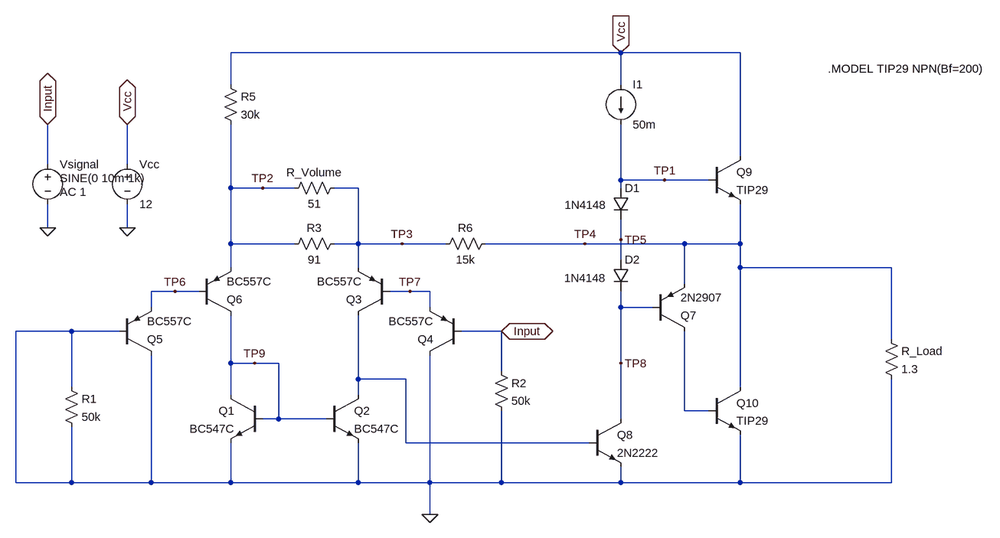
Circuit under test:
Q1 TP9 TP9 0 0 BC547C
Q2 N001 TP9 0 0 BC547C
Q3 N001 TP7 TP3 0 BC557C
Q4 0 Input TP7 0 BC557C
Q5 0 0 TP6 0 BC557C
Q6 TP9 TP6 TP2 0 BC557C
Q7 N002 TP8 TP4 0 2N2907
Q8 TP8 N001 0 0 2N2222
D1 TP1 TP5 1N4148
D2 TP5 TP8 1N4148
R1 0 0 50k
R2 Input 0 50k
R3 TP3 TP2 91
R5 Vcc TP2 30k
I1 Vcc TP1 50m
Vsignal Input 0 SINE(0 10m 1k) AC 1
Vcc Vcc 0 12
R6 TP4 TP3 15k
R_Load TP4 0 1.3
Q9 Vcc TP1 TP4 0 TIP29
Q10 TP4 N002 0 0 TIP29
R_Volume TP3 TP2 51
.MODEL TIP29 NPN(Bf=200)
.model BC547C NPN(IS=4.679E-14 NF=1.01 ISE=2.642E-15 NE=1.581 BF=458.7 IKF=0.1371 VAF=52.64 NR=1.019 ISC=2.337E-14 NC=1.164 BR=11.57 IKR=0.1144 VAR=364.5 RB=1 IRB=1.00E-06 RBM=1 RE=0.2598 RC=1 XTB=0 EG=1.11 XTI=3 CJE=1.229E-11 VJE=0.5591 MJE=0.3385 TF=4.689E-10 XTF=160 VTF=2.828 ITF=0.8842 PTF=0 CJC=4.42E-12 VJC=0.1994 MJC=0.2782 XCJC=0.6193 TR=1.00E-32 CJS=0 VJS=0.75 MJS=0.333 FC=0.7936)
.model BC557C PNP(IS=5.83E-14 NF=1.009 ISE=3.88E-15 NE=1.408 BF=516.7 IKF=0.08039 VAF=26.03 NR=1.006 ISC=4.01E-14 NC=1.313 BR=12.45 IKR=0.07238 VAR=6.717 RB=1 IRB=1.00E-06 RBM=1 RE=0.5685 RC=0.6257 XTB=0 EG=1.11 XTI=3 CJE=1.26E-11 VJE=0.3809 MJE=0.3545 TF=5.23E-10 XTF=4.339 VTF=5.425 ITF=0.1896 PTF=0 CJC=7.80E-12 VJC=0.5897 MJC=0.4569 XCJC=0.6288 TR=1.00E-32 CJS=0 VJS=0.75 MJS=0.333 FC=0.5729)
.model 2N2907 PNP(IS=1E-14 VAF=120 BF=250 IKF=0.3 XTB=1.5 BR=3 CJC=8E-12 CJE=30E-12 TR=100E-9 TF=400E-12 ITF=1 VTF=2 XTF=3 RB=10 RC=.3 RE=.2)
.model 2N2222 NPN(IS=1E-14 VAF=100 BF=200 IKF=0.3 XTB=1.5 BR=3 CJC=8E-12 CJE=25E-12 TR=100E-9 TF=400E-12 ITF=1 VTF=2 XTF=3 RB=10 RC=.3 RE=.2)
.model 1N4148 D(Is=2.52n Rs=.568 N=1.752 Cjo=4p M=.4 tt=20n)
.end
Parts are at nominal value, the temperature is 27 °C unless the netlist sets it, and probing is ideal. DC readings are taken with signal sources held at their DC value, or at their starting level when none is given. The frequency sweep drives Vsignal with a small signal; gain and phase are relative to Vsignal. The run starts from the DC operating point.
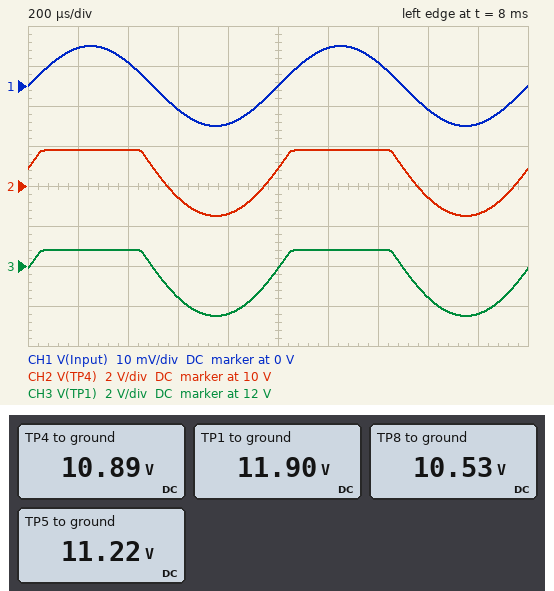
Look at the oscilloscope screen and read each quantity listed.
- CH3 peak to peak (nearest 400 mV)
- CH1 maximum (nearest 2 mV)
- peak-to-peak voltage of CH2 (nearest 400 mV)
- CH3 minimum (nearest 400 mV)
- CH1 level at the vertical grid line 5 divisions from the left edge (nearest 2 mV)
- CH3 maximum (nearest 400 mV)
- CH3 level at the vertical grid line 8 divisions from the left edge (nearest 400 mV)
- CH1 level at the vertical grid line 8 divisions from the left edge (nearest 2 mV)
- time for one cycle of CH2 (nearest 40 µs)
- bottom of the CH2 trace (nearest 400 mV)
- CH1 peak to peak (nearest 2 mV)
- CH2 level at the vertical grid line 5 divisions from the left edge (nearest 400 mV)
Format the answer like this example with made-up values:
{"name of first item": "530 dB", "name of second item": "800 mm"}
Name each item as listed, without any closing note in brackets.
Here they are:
{"CH3 peak to peak": "3.2 V", "CH1 maximum": "10 mV", "peak-to-peak voltage of CH2": "3.2 V", "CH3 minimum": "9.6 V", "CH1 level at the vertical grid line 5 divisions from the left edge": "0 V", "CH3 maximum": "12.8 V", "CH3 level at the vertical grid line 8 divisions from the left edge": "10.4 V", "CH1 level at the vertical grid line 8 divisions from the left edge": "-6 mV", "time for one cycle of CH2": "1.00 ms", "bottom of the CH2 trace": "8.4 V", "CH1 peak to peak": "20 mV", "CH2 level at the vertical grid line 5 divisions from the left edge": "10.8 V"}
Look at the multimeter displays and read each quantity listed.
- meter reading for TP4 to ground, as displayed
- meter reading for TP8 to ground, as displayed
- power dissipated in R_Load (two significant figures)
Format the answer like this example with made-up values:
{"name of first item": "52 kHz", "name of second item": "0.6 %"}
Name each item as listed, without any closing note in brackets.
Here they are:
{"meter reading for TP4 to ground, as displayed": "10.89 V", "meter reading for TP8 to ground, as displayed": "10.53 V", "power dissipated in R_Load": "91 W"}
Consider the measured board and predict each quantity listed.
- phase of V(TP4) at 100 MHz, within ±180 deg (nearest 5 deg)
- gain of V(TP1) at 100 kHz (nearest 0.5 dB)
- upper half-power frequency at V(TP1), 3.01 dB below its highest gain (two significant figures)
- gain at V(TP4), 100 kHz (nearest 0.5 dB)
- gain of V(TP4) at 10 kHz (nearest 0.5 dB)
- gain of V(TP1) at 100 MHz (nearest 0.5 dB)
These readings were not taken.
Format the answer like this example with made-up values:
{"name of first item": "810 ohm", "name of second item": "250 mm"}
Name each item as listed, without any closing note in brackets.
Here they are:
{"phase of V(TP4) at 100 MHz, within ±180 deg": "-165 deg", "gain of V(TP1) at 100 kHz": "45.5 dB", "upper half-power frequency at V(TP1), 3.01 dB below its highest gain": "92 kHz", "gain at V(TP4), 100 kHz": "45.5 dB", "gain of V(TP4) at 10 kHz": "48.5 dB", "gain of V(TP1) at 100 MHz": "4.0 dB"}
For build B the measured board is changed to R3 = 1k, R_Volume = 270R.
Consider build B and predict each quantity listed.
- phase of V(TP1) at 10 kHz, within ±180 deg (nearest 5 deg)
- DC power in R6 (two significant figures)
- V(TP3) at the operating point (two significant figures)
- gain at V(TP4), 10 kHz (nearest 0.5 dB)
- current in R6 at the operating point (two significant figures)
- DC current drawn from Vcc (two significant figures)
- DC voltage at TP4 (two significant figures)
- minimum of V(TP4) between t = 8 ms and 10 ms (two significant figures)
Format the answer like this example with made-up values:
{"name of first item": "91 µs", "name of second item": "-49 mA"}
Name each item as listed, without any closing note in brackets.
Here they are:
{"phase of V(TP1) at 10 kHz, within ±180 deg": "0 deg", "DC power in R6": "4.2 mW", "V(TP3) at the operating point": "1.0 V", "gain at V(TP4), 10 kHz": "38.0 dB", "current in R6 at the operating point": "530 µA", "DC current drawn from Vcc": "6.9 A", "DC voltage at TP4": "9.0 V", "minimum of V(TP4) between t = 8 ms and 10 ms": "8.2 V"}
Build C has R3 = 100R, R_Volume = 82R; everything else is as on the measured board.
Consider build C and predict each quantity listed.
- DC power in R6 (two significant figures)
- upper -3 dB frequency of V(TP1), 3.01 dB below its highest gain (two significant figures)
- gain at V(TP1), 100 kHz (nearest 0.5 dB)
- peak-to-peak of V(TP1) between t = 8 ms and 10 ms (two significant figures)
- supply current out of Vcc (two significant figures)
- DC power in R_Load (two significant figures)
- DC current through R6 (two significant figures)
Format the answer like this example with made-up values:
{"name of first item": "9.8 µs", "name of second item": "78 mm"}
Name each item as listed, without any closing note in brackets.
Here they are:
{"DC power in R6": "6.0 mW", "upper -3 dB frequency of V(TP1), 3.01 dB below its highest gain": "110 kHz", "gain at V(TP1), 100 kHz": "44.5 dB", "peak-to-peak of V(TP1) between t = 8 ms and 10 ms": "3.4 V", "supply current out of Vcc": "8.1 A", "DC power in R_Load": "85 W", "DC current through R6": "630 µA"}
